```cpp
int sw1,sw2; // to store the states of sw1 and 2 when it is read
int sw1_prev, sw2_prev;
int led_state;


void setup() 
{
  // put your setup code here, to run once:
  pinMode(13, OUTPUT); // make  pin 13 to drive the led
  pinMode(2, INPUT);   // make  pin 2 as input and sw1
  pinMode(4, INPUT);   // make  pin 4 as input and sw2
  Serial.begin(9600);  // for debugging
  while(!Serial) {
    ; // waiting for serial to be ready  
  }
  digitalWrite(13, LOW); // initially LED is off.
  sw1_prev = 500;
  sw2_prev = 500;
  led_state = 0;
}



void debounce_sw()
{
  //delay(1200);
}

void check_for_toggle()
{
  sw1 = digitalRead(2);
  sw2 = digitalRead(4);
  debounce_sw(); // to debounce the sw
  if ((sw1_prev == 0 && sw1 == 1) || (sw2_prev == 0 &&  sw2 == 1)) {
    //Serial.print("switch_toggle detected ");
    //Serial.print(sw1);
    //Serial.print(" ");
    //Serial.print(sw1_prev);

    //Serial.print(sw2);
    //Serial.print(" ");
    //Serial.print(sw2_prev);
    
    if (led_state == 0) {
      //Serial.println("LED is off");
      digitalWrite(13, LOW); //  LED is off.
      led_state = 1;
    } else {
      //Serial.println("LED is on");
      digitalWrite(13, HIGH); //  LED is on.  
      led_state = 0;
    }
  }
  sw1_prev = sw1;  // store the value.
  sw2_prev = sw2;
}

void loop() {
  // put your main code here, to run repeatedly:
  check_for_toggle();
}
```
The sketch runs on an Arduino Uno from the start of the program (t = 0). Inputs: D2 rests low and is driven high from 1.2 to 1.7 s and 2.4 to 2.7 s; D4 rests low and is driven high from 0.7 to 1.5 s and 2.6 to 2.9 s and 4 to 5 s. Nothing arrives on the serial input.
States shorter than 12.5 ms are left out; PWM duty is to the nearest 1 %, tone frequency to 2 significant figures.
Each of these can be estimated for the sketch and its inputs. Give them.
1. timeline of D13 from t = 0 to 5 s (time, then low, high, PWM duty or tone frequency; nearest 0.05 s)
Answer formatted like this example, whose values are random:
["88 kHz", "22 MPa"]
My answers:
["0 s low; 1.2 s high; 2.4 s low; 2.6 s high; 4 s low"]
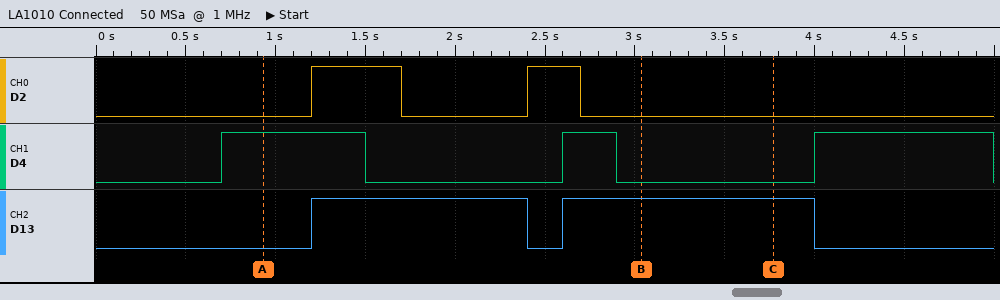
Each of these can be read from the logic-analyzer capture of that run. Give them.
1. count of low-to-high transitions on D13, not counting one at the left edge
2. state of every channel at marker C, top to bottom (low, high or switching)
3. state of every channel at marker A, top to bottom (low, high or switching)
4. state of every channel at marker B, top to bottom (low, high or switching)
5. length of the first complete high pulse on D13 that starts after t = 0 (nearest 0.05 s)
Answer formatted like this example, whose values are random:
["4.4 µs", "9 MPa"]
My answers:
["2", "D2 low, D4 low, D13 high", "D2 low, D4 high, D13 low", "D2 low, D4 low, D13 high", "1.20 s"]
